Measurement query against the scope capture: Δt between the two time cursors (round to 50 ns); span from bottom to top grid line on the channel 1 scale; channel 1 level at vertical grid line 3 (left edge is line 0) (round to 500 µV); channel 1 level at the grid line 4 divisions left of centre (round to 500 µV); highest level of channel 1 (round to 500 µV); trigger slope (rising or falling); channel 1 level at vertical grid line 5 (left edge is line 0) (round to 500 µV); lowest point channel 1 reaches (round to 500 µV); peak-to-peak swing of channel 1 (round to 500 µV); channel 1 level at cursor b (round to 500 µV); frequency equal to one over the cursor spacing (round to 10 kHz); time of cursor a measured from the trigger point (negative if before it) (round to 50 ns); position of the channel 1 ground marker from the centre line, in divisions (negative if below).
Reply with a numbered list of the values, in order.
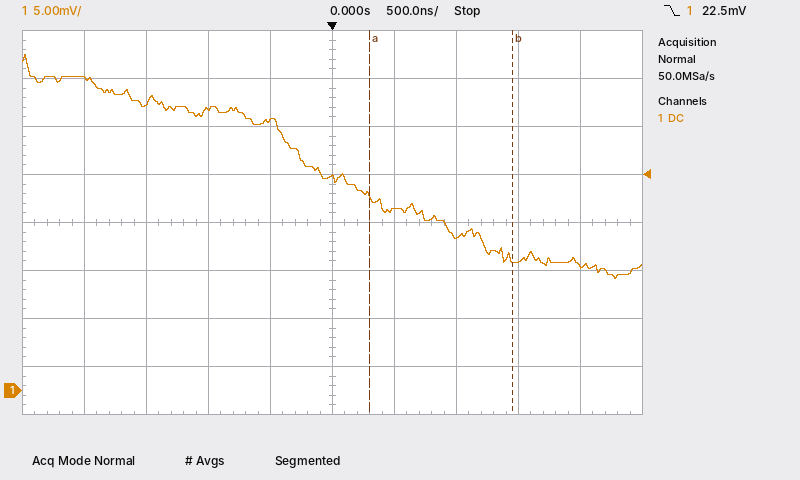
1. 1.15 µs
2. 40 mV
3. 29.5 mV
4. 32.5 mV
5. 35.0 mV
6. falling
7. 22.0 mV
8. 11.5 mV
9. 23.5 mV
10. 14.0 mV
11. 870 kHz
12. +300 ns
13. -3.5 div
